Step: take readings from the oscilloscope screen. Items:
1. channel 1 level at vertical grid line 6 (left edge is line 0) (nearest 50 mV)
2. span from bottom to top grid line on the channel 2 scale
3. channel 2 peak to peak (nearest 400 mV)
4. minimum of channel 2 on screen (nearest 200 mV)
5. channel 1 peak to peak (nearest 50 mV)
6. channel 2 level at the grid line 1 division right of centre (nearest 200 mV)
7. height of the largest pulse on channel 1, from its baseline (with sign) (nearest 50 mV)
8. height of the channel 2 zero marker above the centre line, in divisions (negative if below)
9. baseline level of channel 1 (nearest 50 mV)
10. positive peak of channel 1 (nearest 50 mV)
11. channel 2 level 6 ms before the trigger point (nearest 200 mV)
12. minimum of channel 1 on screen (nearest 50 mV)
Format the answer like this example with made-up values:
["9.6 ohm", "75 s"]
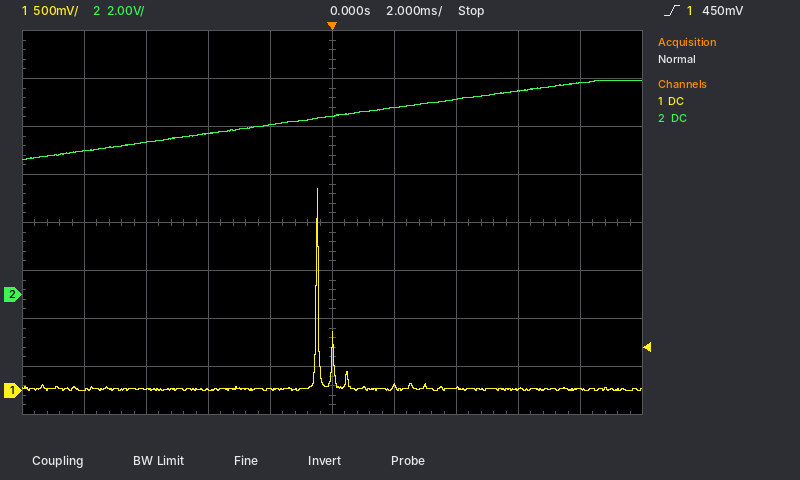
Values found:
["50 mV", "16 V", "3.2 V", "5.6 V", "2.10 V", "7.8 V", "+2.10 V", "-1.5 div", "0 mV", "2.10 V", "6.4 V", "0 mV"]
